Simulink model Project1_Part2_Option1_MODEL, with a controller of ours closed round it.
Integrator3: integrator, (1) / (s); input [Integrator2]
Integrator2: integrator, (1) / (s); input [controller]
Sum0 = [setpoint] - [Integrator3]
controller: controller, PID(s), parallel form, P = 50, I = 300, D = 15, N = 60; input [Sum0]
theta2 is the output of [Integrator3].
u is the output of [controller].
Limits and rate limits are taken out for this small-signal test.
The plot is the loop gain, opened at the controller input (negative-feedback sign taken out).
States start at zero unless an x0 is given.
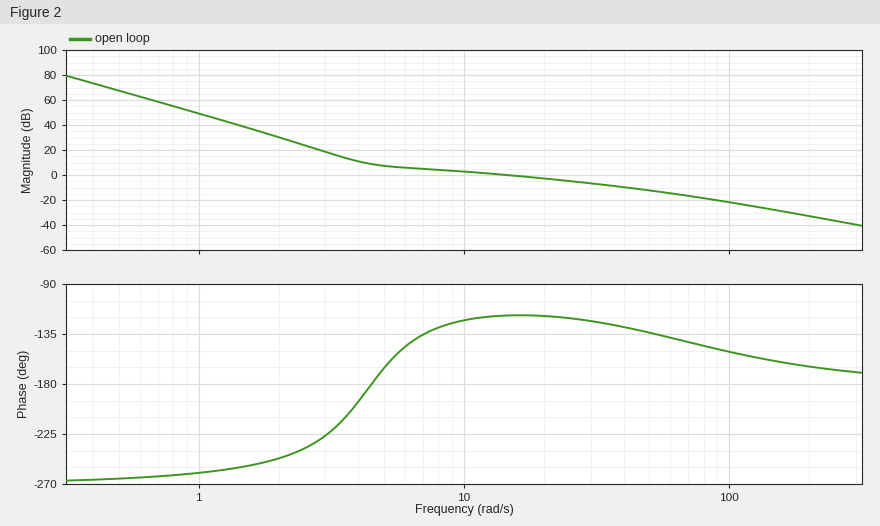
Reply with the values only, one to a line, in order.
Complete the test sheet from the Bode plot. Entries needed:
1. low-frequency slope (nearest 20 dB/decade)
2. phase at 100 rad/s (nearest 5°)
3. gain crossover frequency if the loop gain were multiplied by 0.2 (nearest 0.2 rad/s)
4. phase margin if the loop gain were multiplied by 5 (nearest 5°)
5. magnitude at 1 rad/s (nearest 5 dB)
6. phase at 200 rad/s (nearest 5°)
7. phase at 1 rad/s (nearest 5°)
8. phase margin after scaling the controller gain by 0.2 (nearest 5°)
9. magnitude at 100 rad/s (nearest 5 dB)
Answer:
-60 dB/decade
-150°
3.6 rad/s
45°
50 dB
-165°
-260°
-30°
-20 dB
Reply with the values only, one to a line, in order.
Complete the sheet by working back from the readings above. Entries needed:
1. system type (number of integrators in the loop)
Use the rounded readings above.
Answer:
3
